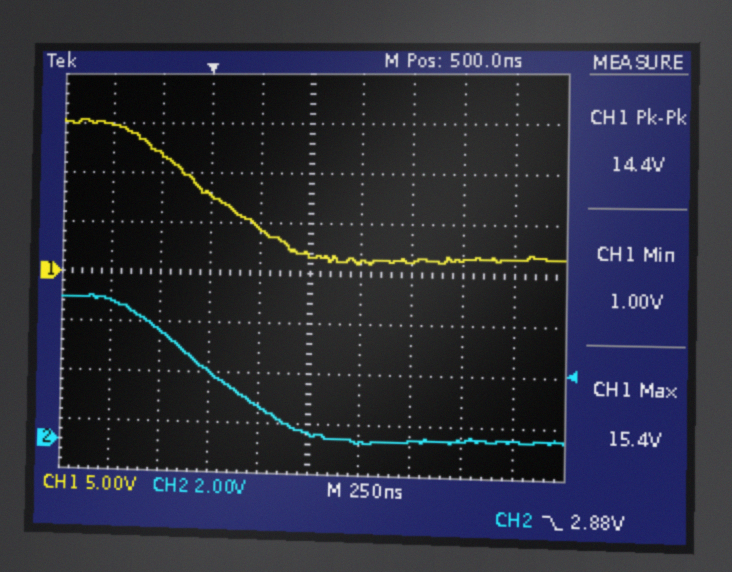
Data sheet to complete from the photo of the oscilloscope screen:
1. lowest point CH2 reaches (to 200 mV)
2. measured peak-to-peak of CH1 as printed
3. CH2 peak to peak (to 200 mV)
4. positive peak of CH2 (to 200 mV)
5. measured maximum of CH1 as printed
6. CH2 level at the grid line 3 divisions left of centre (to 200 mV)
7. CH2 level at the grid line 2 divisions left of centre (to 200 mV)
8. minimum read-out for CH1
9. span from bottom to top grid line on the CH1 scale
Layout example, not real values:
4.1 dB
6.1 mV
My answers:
0.0 V
14.4 V
5.8 V
5.8 V
15.4 V
4.4 V
2.8 V
1.00 V
40 V
